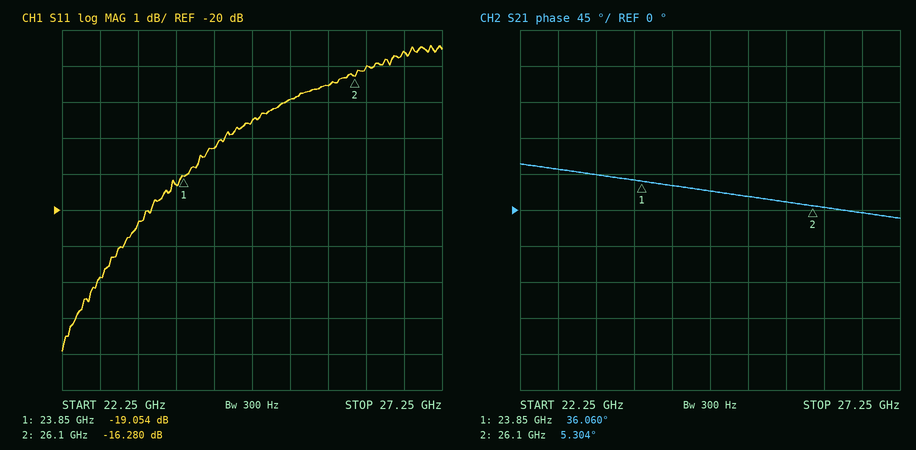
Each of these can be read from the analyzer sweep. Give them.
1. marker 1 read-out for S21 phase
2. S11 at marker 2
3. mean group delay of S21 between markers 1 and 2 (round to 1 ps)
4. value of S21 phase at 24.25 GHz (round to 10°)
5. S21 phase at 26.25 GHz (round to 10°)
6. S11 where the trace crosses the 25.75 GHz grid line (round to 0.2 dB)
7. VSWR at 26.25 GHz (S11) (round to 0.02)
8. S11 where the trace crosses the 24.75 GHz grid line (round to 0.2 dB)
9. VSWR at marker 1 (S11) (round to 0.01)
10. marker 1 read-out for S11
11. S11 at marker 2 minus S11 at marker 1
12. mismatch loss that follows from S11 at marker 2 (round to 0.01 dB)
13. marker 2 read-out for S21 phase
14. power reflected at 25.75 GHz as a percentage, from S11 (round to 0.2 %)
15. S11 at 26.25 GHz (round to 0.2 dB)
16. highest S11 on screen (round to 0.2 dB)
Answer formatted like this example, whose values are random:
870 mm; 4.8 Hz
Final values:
36.060°; -16.280 dB; 38 ps; 30°; 0°; -16.6 dB; 1.38; -17.6 dB; 1.25; -19.054 dB; 2.774 dB; 0.10 dB; 5.304°; 2.2 %; -16.0 dB; -15.4 dB
